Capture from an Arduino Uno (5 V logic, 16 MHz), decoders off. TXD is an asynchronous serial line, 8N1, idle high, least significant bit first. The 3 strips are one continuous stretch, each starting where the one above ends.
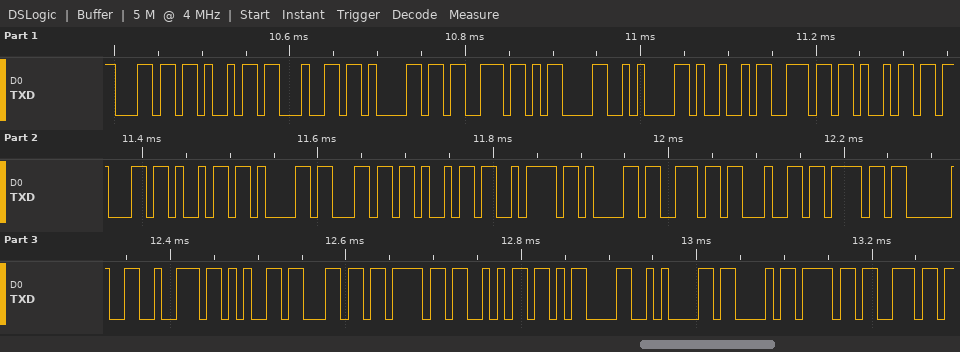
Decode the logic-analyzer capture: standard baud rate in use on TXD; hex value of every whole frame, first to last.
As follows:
115200 baud
0x6C 0x69 0x64 0x61 0x73 0x0D 0x0A 0x49 0x6E 0x69 0x63 0x69 0x61 0x6C 0x69 0x7A 0x61 0x6E 0x64 0x6F 0x20 0x72 0x65 0x6C 0x6F 0x6A 0x0D 0x0A 0x43 0x6F 0x6E
